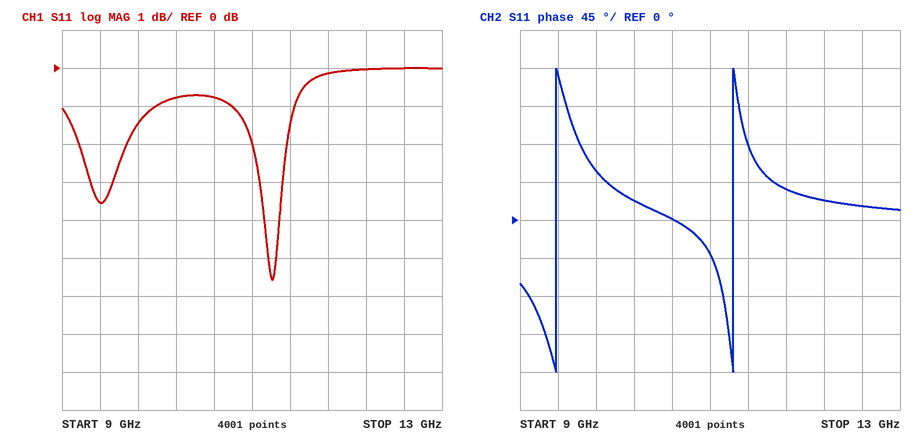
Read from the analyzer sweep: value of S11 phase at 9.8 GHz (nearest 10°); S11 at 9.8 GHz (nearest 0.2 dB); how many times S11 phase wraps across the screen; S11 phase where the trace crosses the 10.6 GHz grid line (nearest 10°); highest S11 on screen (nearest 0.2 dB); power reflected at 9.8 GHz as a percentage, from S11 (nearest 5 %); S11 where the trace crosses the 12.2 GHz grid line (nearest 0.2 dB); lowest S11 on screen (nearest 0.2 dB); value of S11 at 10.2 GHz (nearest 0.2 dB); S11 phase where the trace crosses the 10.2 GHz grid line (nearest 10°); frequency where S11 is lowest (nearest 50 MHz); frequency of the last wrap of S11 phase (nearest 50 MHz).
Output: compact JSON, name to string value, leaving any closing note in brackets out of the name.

{"value of S11 phase at 9.8 GHz": "60°", "S11 at 9.8 GHz": "-1.4 dB", "how many times S11 phase wraps across the screen": "2", "S11 phase where the trace crosses the 10.6 GHz grid line": "0°", "highest S11 on screen": "0.0 dB", "power reflected at 9.8 GHz as a percentage, from S11": "70 %", "S11 where the trace crosses the 12.2 GHz grid line": "0.0 dB", "lowest S11 on screen": "-5.6 dB", "value of S11 at 10.2 GHz": "-0.8 dB", "S11 phase where the trace crosses the 10.2 GHz grid line": "20°", "frequency where S11 is lowest": "11.20 GHz", "frequency of the last wrap of S11 phase": "11.25 GHz"}
